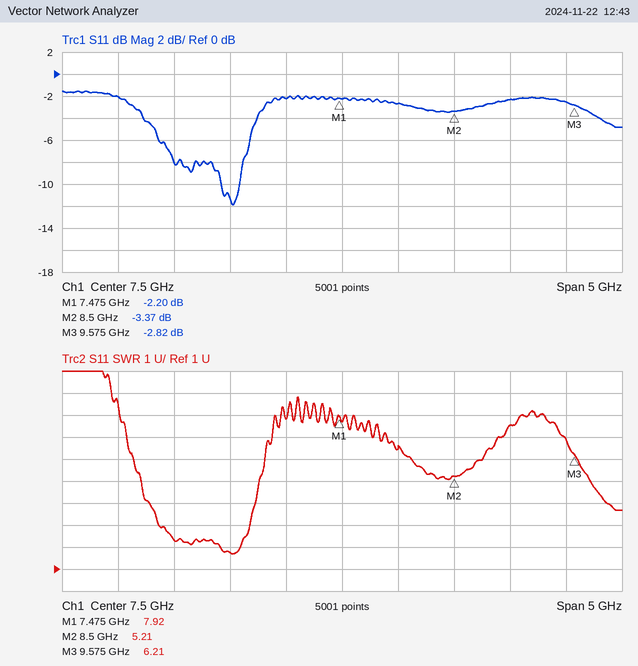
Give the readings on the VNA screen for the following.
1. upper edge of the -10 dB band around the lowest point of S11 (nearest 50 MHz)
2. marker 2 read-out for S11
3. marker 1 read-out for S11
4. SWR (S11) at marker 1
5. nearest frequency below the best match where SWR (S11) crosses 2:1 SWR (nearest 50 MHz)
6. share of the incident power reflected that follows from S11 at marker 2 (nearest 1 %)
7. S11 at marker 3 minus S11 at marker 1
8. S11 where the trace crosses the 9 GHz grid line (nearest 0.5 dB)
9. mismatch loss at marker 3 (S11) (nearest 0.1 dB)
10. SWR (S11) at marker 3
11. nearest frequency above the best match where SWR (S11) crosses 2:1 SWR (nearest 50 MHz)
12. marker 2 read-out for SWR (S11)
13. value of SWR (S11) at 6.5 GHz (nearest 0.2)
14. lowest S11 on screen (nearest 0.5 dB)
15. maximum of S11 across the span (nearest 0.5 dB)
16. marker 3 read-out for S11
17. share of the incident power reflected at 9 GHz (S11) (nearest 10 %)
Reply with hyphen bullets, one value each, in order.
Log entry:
- 6.60 GHz
- -3.37 dB
- -2.20 dB
- 7.92
- 6.40 GHz
- 46 %
- -0.62 dB
- -2.5 dB
- 3.2 dB
- 6.21
- 6.60 GHz
- 5.21
- 1.8
- -12.0 dB
- -1.5 dB
- -2.82 dB
- 60 %
